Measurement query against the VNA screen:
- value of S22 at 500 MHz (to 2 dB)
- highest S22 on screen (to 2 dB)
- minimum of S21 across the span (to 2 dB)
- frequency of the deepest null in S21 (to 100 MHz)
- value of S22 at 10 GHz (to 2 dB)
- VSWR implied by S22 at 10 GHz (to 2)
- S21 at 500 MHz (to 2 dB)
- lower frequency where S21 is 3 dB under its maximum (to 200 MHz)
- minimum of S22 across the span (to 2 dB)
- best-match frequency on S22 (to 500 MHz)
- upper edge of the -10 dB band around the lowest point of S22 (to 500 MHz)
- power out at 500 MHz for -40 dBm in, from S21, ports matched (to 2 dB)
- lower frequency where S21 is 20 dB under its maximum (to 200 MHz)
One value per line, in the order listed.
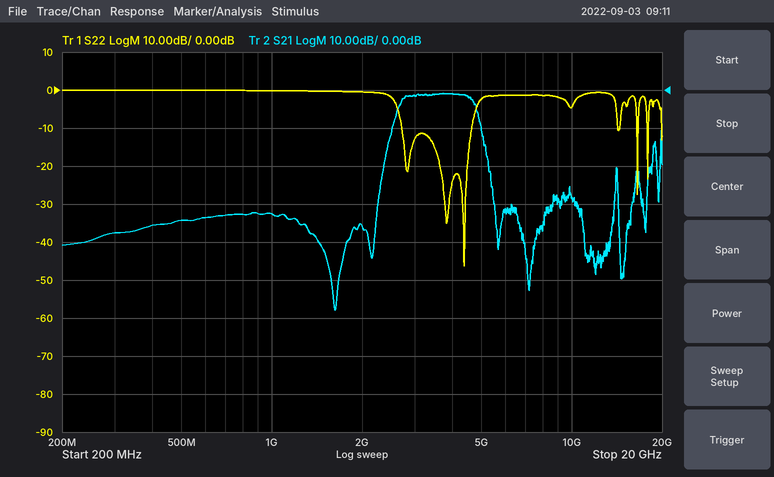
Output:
0 dB
0 dB
-58 dB
1.6 GHz
-4 dB
4
-34 dB
2.6 GHz
-46 dB
4.5 GHz
4.5 GHz
-74 dBm
2.4 GHz
